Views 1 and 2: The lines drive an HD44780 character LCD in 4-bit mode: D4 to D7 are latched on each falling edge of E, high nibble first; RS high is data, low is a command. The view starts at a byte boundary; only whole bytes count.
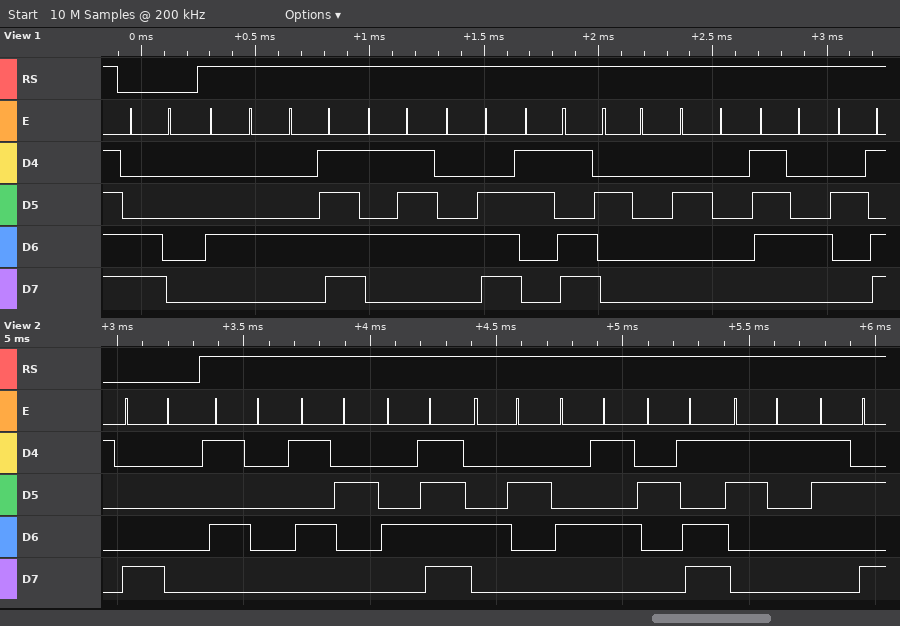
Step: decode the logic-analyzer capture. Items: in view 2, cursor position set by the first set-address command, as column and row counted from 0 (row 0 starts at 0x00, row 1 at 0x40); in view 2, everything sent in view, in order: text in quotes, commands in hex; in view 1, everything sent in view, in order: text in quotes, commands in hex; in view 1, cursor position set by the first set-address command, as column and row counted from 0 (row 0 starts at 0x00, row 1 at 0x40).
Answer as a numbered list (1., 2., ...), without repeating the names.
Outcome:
1. column 0, row 0
2. 0x80 "PROBE-1:"
3. 0xC0 "DOWN=  t-"
4. column 0, row 1
